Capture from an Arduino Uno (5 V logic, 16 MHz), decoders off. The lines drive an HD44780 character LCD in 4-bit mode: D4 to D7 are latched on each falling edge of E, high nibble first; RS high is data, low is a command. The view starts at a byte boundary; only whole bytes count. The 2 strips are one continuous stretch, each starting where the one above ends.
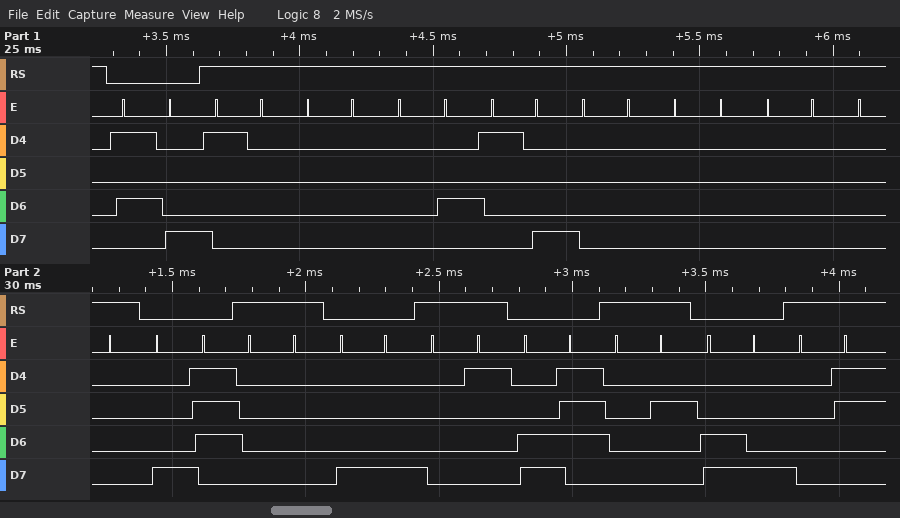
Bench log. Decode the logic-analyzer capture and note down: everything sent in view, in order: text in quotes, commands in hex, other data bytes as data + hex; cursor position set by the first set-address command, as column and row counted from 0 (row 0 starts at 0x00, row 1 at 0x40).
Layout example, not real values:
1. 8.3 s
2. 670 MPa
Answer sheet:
1. 0x58 data 10 00 04 18 00 00 00 00 0x87 data 00 0x88 data 01 0xC7 data 02 0xC8 data 03
2. column 7, row 0
